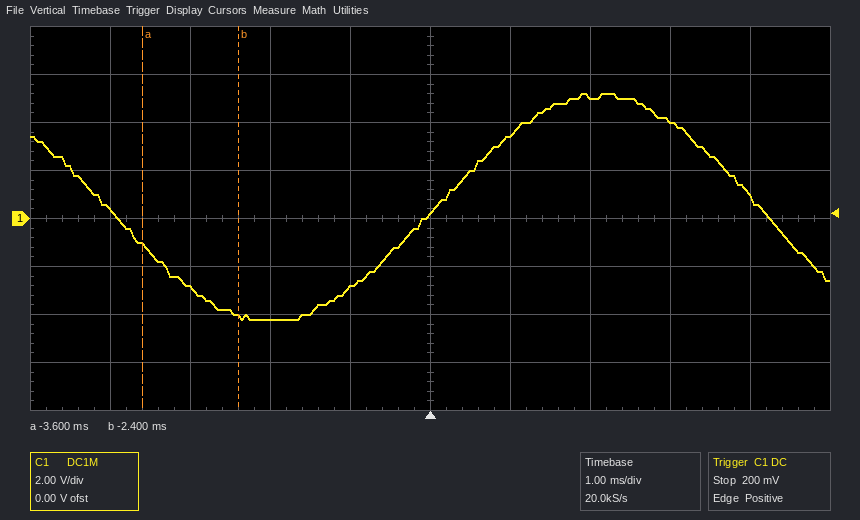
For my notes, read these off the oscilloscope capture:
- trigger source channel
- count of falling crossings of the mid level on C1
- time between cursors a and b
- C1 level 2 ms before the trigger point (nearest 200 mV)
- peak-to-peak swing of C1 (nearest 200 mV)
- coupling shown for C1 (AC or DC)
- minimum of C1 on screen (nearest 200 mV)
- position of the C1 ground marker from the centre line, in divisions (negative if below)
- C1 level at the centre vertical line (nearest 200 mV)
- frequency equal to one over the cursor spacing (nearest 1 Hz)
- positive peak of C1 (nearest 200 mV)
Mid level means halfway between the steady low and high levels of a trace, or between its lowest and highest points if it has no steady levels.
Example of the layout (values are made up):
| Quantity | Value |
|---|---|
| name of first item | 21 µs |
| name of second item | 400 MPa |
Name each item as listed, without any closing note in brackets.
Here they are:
| Quantity | Value |
|---|---|
| trigger source channel | C1 |
| count of falling crossings of the mid level on C1 | 2 |
| time between cursors a and b | 1.2 ms |
| C1 level 2 ms before the trigger point | -4.2 V |
| peak-to-peak swing of C1 | 9.4 V |
| coupling shown for C1 | DC |
| minimum of C1 on screen | -4.2 V |
| position of the C1 ground marker from the centre line, in divisions | 0.0 div |
| C1 level at the centre vertical line | 200 mV |
| frequency equal to one over the cursor spacing | 833 Hz |
| positive peak of C1 | 5.2 V |
